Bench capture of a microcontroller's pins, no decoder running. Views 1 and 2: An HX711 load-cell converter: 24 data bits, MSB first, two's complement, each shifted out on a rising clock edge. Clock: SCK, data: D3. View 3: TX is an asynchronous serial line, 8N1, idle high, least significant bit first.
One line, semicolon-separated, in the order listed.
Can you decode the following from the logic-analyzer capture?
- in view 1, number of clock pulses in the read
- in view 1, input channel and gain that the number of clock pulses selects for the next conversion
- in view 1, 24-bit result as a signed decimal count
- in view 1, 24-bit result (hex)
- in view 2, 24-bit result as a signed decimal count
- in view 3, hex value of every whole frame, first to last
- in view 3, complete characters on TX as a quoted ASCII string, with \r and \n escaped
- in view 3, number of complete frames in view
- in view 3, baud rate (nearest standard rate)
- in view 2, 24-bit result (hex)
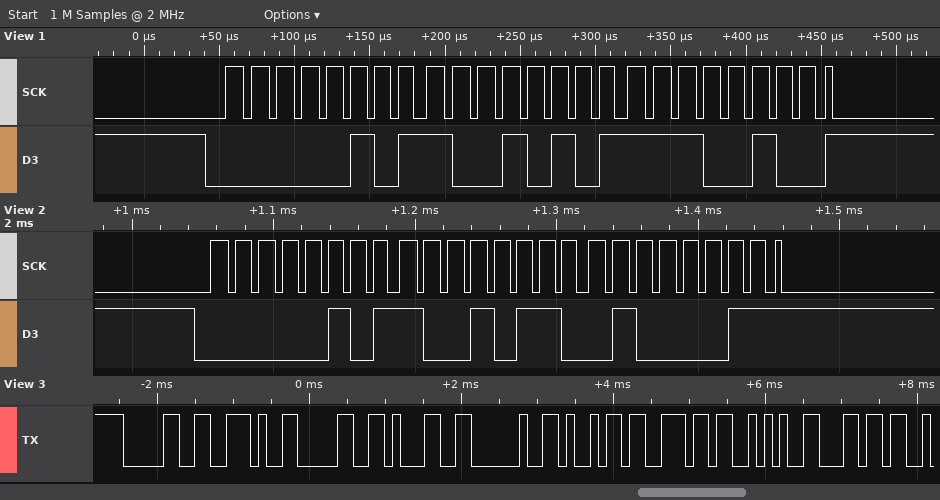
25; channel A, gain 128; 366052; 0x0595E4; 366147; 30 2E 30 31 20 69 6E 2A 6C; "0.01 in*l"; 9; 9600 baud; 0x059643
